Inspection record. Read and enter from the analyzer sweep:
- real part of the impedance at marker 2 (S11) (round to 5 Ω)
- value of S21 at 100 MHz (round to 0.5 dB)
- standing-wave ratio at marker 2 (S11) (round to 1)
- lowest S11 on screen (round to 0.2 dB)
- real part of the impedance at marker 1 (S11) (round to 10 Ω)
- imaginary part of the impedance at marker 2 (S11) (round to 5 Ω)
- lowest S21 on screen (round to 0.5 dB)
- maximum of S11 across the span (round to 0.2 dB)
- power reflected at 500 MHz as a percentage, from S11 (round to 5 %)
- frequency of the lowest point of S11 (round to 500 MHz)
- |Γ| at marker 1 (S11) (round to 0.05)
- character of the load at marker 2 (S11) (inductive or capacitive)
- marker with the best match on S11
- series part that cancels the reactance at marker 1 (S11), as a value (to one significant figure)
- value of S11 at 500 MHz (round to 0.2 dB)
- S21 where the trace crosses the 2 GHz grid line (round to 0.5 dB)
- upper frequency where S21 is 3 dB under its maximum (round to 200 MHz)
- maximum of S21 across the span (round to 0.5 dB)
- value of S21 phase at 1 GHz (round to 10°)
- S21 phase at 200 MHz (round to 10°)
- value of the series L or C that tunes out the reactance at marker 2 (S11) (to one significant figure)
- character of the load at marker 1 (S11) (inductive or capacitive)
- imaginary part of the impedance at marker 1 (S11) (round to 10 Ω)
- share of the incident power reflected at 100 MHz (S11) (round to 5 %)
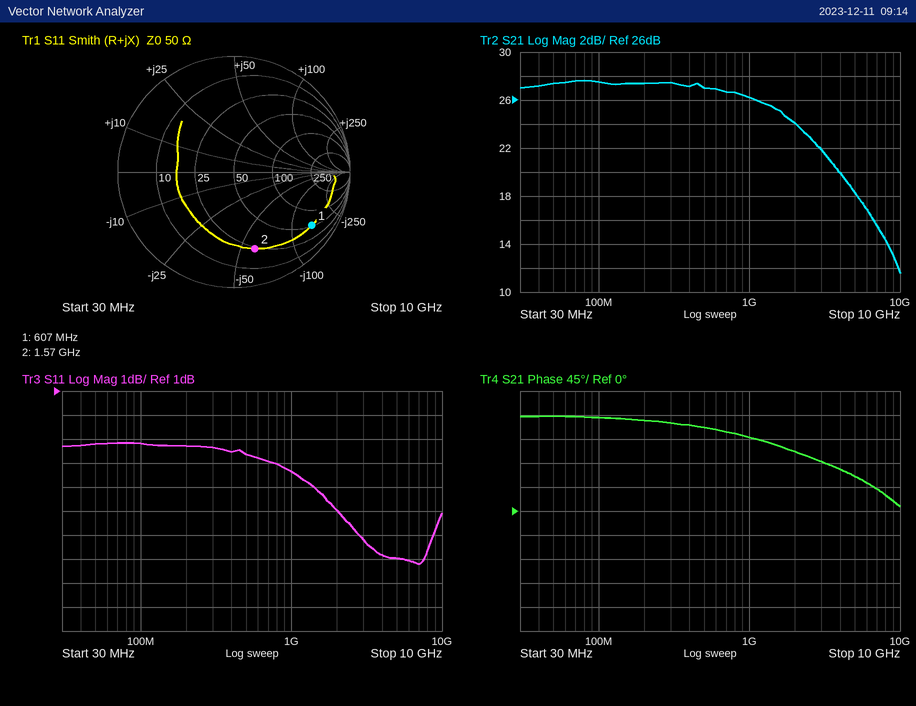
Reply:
25 Ω
27.5 dB
5
-6.2 dB
50 Ω
-60 Ω
11.5 dB
-1.2 dB
70 %
7.0 GHz
0.80
capacitive
marker 2
40 nH
-1.6 dB
24.0 dB
1.8 GHz
27.5 dB
140°
170°
6 nH
capacitive
-140 Ω
75 %
